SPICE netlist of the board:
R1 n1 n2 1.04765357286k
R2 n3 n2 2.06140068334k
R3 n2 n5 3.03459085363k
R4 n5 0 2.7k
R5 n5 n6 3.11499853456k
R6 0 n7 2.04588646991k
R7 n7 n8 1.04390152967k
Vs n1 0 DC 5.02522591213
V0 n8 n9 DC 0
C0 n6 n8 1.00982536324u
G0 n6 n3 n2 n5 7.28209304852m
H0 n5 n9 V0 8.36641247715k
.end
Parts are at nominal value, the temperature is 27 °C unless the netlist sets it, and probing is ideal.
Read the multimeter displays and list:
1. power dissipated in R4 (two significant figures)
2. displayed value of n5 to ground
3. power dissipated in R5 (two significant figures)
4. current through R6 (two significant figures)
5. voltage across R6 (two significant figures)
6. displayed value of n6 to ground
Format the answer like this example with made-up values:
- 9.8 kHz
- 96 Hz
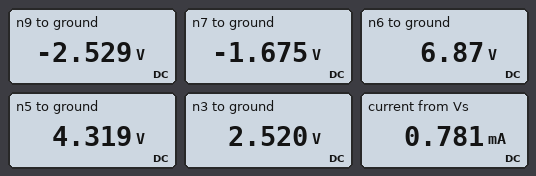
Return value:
- 6.9 mW
- 4.319 V
- 2.1 mW
- 820 µA
- 1.7 V
- 6.87 V
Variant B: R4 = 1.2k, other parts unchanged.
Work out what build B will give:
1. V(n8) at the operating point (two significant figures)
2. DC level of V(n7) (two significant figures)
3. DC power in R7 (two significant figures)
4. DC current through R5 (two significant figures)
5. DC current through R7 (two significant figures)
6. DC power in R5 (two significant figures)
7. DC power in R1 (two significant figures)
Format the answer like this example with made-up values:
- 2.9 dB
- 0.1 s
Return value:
- -1.9 V
- -1.2 V
- 380 µW
- 2.1 mA
- 600 µA
- 14 mW
- 4.4 mW
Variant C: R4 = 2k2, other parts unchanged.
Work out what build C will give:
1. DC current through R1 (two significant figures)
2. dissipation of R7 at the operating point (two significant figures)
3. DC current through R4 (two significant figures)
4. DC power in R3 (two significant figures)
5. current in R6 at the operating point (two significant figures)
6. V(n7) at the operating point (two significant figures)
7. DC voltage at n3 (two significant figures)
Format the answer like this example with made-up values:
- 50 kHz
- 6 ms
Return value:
- 1.1 mA
- 620 µW
- 1.8 mA
- 7.9 µW
- 770 µA
- -1.6 V
- 1.6 V
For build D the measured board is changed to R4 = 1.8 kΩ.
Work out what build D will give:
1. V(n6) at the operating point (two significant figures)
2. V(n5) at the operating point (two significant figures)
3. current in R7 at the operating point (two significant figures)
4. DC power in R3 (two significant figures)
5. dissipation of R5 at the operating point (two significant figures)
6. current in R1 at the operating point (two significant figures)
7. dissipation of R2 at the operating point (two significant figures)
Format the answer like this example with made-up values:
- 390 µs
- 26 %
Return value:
- 8.3 V
- 3.8 V
- 720 µA
- 13 µW
- 6.5 mW
- 1.4 mA
- 4.3 mW
